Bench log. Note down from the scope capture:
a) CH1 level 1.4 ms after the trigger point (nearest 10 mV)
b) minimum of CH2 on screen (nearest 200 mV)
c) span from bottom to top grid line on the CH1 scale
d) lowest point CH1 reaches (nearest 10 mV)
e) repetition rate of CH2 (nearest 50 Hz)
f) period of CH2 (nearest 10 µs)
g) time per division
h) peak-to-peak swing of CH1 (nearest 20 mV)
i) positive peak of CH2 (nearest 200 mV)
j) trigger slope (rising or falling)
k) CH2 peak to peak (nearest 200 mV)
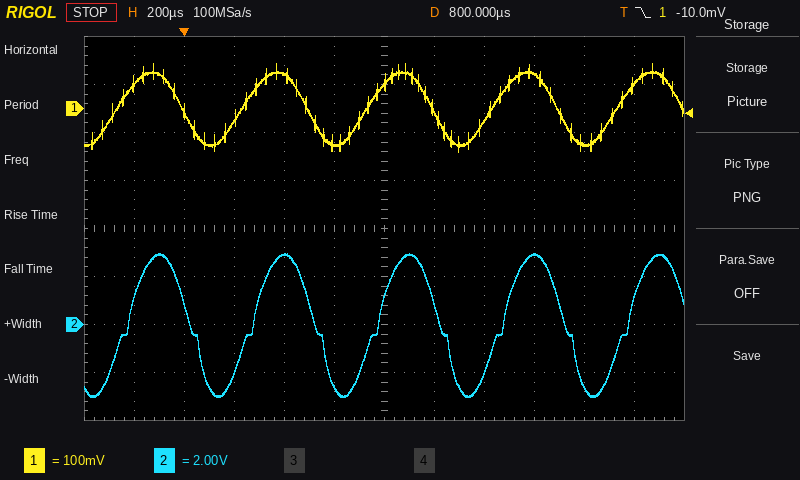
70 mV
-3.0 V
800 mV
-90 mV
2.00 kHz
500 µs
200 µs
180 mV
3.0 V
falling
6.0 V
